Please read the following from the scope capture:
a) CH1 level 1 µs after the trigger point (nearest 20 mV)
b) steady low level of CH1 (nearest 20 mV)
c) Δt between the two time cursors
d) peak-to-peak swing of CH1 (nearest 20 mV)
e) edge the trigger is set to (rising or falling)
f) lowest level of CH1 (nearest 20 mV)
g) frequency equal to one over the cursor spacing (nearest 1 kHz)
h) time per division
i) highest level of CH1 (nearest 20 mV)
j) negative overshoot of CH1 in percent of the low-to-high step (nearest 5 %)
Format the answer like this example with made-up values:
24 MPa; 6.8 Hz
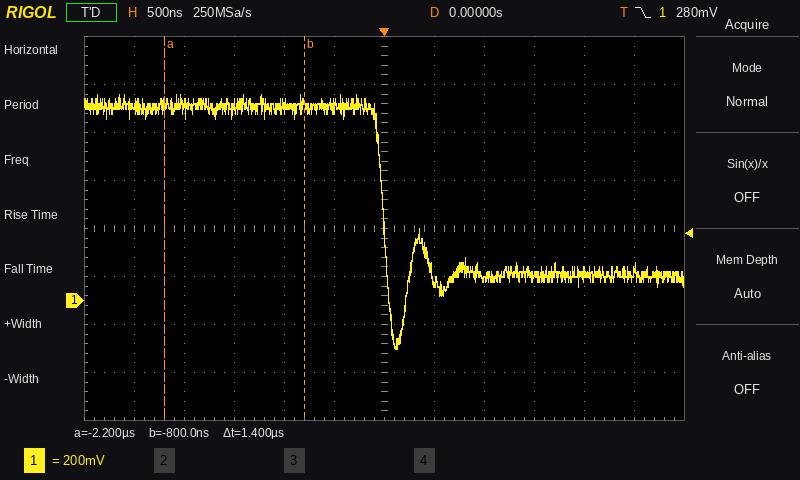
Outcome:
100 mV; 100 mV; 1.4 µs; 1.06 V; falling; -200 mV; 714 kHz; 500 ns; 860 mV; 45 %
